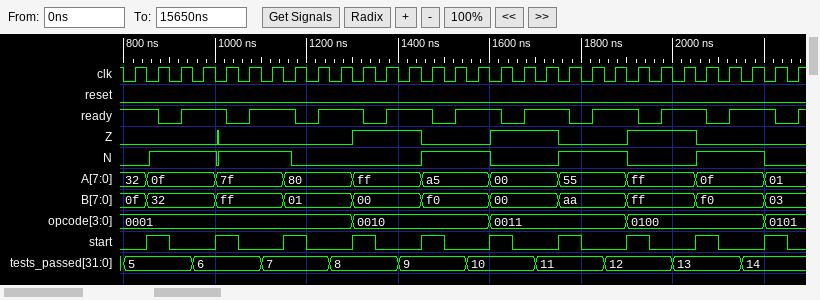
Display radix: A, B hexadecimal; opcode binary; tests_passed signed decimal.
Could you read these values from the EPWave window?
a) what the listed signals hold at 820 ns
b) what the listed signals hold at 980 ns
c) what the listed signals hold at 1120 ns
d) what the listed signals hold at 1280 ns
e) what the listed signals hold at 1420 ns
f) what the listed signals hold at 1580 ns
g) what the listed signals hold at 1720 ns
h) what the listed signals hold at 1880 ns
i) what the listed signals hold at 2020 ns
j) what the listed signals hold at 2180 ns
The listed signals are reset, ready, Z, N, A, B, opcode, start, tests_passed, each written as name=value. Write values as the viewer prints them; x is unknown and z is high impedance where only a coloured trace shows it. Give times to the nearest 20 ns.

reset=0, ready=1, Z=0, N=0, A=32, B=0f, opcode=0001, start=0, tests_passed=5
reset=0, ready=1, Z=0, N=1, A=0f, B=32, opcode=0001, start=0, tests_passed=6
reset=0, ready=1, Z=0, N=1, A=7f, B=ff, opcode=0001, start=0, tests_passed=7
reset=0, ready=1, Z=0, N=0, A=80, B=01, opcode=0001, start=0, tests_passed=8
reset=0, ready=1, Z=1, N=0, A=ff, B=00, opcode=0010, start=0, tests_passed=9
reset=0, ready=1, Z=0, N=1, A=a5, B=f0, opcode=0010, start=0, tests_passed=10
reset=0, ready=1, Z=1, N=0, A=00, B=00, opcode=0011, start=0, tests_passed=11
reset=0, ready=1, Z=0, N=1, A=55, B=aa, opcode=0011, start=0, tests_passed=12
reset=0, ready=1, Z=1, N=0, A=ff, B=ff, opcode=0100, start=0, tests_passed=13
reset=0, ready=1, Z=0, N=1, A=0f, B=f0, opcode=0100, start=0, tests_passed=14
